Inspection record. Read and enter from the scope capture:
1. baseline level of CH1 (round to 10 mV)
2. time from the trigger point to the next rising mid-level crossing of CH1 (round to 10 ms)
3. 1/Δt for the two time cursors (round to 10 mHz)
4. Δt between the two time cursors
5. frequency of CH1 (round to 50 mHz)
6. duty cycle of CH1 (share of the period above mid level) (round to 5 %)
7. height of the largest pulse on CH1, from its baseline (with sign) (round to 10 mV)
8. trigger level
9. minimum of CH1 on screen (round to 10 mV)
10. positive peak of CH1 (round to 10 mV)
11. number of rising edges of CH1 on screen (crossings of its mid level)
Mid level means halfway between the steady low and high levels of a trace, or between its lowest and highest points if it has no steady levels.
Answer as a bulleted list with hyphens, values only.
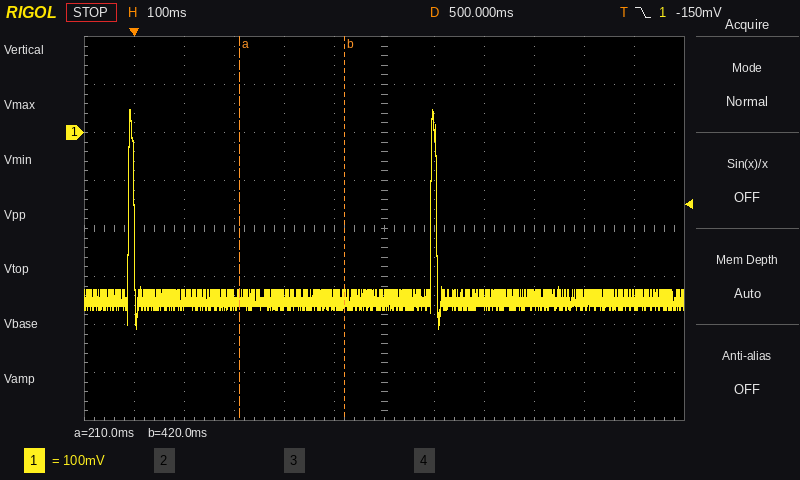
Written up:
- -350 mV
- 590 ms
- 4.76 Hz
- 210 ms
- 1.65 Hz
- 0 %
- +400 mV
- -150 mV
- -410 mV
- 50 mV
- 2
